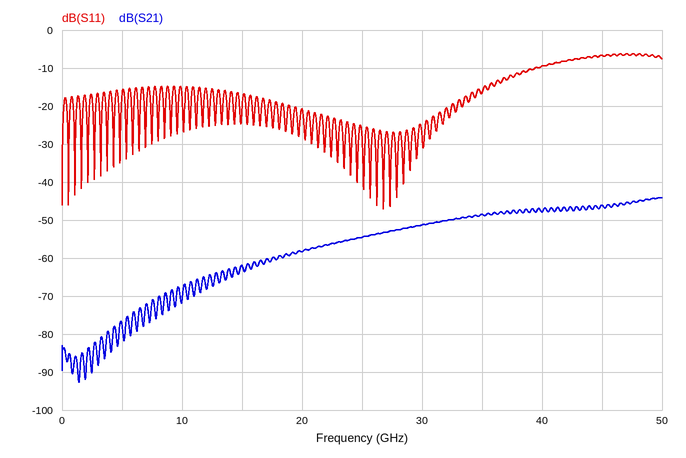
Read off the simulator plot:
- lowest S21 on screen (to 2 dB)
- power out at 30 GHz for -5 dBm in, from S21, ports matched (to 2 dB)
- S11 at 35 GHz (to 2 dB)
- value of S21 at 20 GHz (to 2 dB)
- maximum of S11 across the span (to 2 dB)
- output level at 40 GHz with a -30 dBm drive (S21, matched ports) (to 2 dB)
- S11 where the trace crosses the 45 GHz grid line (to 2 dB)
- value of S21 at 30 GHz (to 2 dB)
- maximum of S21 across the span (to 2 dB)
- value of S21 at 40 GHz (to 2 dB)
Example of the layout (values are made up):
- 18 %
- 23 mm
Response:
- -92 dB
- -56 dBm
- -16 dB
- -58 dB
- -6 dB
- -78 dBm
- -6 dB
- -52 dB
- -44 dB
- -48 dB
